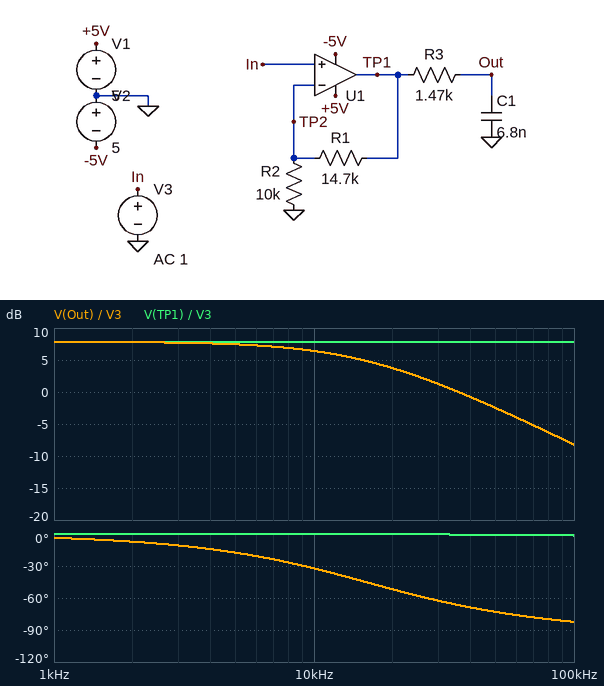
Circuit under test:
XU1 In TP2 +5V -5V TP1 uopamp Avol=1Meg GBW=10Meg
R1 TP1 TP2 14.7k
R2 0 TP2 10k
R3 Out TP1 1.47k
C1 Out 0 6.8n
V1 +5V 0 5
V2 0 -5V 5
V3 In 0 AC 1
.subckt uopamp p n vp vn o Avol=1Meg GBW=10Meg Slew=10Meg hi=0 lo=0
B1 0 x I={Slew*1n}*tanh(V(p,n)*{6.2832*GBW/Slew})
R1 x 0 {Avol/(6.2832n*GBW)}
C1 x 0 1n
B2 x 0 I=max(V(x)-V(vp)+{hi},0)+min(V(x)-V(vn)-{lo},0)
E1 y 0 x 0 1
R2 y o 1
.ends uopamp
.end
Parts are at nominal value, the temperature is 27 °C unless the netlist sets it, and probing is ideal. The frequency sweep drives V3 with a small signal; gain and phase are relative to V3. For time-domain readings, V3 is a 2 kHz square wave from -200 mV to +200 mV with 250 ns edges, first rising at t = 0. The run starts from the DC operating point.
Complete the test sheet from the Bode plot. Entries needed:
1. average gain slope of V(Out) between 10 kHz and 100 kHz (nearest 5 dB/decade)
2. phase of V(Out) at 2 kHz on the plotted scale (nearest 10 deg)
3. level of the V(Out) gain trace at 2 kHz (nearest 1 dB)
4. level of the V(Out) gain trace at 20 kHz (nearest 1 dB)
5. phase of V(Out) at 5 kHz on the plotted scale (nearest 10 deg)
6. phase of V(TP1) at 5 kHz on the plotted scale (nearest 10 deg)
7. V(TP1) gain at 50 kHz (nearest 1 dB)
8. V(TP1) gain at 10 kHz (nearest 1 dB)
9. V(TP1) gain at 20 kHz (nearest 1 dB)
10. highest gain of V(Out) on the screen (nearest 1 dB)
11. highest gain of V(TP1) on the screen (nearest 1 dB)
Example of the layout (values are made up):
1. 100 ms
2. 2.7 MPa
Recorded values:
1. -15 dB/decade
2. -10 deg
3. 8 dB
4. 4 dB
5. -20 deg
6. 0 deg
7. 8 dB
8. 8 dB
9. 8 dB
10. 8 dB
11. 8 dB
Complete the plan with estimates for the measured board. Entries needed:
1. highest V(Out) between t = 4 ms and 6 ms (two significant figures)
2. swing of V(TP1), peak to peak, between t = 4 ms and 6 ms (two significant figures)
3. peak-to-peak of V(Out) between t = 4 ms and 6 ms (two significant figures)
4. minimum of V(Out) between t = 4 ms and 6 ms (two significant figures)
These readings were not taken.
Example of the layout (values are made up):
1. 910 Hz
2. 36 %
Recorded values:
1. 490 mV
2. 990 mV
3. 990 mV
4. -490 mV
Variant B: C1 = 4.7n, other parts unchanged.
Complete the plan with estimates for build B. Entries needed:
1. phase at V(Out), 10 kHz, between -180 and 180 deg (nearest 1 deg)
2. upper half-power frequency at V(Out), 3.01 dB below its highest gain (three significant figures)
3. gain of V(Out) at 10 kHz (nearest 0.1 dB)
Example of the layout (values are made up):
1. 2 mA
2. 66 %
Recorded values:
1. -24 deg
2. 23.0 kHz
3. 7.1 dB
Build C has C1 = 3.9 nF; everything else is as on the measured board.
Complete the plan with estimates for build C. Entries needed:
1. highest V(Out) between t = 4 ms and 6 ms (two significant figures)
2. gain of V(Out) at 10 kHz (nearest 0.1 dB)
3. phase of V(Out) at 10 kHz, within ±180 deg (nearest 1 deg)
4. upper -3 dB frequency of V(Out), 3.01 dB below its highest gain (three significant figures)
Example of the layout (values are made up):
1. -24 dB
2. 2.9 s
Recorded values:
1. 490 mV
2. 7.3 dB
3. -20 deg
4. 27.8 kHz
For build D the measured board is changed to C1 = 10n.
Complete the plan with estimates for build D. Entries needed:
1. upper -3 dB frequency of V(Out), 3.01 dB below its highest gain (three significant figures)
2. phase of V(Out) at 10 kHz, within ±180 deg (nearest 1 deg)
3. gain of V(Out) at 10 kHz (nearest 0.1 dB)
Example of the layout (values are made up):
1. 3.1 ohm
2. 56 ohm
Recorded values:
1. 10.8 kHz
2. -43 deg
3. 5.2 dB
